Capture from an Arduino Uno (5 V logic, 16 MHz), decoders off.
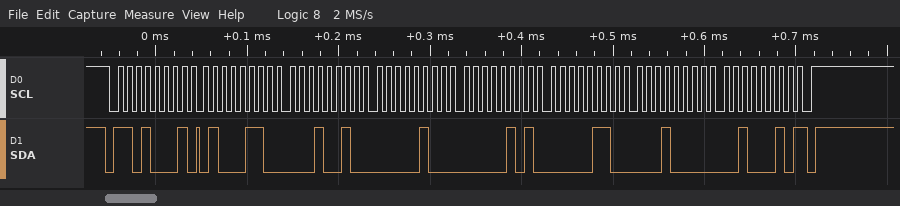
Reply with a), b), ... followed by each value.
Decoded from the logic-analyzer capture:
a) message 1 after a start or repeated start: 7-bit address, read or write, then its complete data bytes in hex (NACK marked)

a) 0x68 read: 46 12 04 05 06 10 22 NACK
